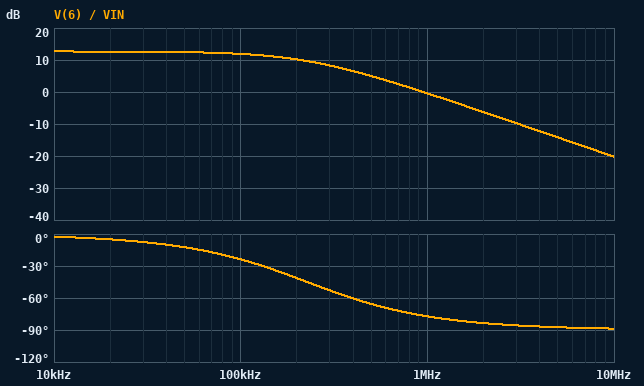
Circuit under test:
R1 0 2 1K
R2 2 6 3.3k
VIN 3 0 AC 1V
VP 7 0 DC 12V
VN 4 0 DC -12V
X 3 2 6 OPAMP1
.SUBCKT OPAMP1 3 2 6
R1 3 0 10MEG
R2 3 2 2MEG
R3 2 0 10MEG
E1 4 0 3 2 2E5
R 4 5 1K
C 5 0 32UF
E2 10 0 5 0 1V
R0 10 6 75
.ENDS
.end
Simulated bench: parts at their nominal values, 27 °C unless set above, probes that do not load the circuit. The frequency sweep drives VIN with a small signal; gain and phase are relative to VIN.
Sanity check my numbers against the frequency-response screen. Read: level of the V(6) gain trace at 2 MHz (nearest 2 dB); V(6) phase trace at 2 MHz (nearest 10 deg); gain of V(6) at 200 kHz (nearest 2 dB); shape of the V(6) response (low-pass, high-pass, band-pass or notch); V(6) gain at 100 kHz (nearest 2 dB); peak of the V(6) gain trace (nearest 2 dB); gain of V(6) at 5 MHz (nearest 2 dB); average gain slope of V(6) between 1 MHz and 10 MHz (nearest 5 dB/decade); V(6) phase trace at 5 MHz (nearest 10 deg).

-6 dB
-80 deg
10 dB
low-pass
12 dB
12 dB
-14 dB
-20 dB/decade
-90 deg
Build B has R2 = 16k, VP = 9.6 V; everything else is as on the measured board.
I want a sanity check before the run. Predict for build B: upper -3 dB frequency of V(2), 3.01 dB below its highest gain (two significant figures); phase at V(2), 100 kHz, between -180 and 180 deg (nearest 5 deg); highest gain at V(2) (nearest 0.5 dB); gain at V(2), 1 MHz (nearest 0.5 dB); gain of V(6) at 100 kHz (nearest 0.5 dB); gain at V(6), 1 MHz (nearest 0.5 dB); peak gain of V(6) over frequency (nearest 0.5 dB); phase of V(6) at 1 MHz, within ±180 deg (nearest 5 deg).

58 kHz
-60 deg
0 dB
-24.5 dB
18.5 dB
0 dB
24.5 dB
-85 deg
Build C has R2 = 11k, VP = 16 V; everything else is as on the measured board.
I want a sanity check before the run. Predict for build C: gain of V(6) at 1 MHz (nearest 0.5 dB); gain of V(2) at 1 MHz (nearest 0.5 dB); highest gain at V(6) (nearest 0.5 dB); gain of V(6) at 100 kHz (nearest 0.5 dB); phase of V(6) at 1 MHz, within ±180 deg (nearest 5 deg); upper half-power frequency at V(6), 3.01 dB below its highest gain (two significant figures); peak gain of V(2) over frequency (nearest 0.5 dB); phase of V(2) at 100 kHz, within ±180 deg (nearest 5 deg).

0 dB
-21.5 dB
21.5 dB
17.5 dB
-85 deg
82 kHz
0 dB
-50 deg
